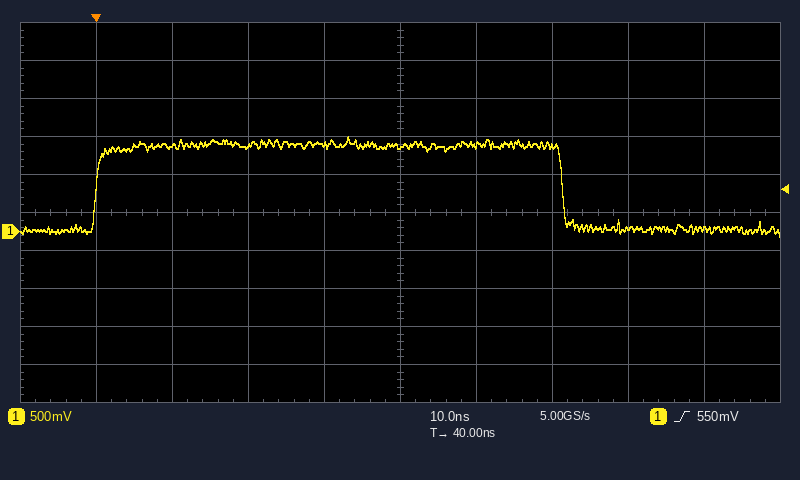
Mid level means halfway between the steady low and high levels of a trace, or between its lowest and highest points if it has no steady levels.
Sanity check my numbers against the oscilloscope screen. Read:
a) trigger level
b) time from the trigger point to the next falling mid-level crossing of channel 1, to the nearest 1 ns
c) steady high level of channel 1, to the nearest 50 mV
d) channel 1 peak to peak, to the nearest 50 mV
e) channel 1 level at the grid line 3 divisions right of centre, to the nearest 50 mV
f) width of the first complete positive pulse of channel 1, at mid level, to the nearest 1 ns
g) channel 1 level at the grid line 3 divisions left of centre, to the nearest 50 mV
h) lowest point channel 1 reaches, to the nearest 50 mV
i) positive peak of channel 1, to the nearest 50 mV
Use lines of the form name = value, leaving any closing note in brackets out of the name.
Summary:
trigger level = 550 mV
time from the trigger point to the next falling mid-level crossing of channel 1, to the nearest 1 ns = 61 ns
steady high level of channel 1, to the nearest 50 mV = 1.15 V
channel 1 peak to peak, to the nearest 50 mV = 1.30 V
channel 1 level at the grid line 3 divisions right of centre, to the nearest 50 mV = 50 mV
width of the first complete positive pulse of channel 1, at mid level, to the nearest 1 ns = 61 ns
channel 1 level at the grid line 3 divisions left of centre, to the nearest 50 mV = 1.10 V
lowest point channel 1 reaches, to the nearest 50 mV = -50 mV
positive peak of channel 1, to the nearest 50 mV = 1.25 V
